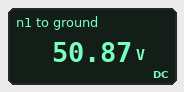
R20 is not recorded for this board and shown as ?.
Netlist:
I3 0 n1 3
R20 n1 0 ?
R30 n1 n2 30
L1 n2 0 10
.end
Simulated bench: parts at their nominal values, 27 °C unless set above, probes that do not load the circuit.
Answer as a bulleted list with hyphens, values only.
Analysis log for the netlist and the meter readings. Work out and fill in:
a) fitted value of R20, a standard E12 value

- 39 Ω
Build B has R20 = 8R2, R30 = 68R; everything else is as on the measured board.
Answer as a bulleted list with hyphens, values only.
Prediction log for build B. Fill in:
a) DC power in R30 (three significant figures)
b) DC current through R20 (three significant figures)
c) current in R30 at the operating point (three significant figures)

- 7.09 W
- 2.68 A
- 323 mA
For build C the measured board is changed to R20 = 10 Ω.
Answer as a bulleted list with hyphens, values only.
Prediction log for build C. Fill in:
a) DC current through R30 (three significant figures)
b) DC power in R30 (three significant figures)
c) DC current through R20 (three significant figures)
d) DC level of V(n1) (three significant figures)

- 750 mA
- 16.9 W
- 2.25 A
- 22.5 V
